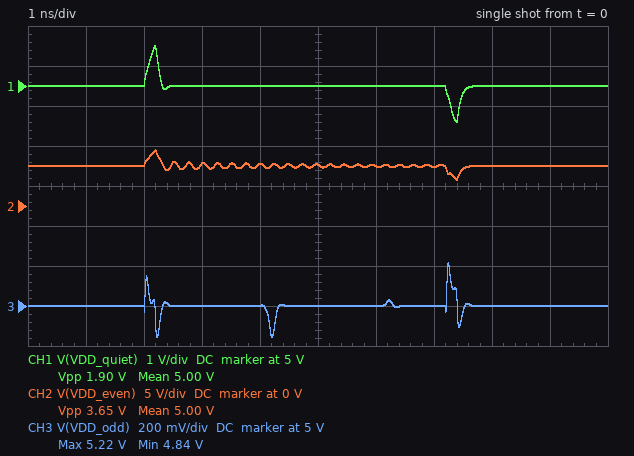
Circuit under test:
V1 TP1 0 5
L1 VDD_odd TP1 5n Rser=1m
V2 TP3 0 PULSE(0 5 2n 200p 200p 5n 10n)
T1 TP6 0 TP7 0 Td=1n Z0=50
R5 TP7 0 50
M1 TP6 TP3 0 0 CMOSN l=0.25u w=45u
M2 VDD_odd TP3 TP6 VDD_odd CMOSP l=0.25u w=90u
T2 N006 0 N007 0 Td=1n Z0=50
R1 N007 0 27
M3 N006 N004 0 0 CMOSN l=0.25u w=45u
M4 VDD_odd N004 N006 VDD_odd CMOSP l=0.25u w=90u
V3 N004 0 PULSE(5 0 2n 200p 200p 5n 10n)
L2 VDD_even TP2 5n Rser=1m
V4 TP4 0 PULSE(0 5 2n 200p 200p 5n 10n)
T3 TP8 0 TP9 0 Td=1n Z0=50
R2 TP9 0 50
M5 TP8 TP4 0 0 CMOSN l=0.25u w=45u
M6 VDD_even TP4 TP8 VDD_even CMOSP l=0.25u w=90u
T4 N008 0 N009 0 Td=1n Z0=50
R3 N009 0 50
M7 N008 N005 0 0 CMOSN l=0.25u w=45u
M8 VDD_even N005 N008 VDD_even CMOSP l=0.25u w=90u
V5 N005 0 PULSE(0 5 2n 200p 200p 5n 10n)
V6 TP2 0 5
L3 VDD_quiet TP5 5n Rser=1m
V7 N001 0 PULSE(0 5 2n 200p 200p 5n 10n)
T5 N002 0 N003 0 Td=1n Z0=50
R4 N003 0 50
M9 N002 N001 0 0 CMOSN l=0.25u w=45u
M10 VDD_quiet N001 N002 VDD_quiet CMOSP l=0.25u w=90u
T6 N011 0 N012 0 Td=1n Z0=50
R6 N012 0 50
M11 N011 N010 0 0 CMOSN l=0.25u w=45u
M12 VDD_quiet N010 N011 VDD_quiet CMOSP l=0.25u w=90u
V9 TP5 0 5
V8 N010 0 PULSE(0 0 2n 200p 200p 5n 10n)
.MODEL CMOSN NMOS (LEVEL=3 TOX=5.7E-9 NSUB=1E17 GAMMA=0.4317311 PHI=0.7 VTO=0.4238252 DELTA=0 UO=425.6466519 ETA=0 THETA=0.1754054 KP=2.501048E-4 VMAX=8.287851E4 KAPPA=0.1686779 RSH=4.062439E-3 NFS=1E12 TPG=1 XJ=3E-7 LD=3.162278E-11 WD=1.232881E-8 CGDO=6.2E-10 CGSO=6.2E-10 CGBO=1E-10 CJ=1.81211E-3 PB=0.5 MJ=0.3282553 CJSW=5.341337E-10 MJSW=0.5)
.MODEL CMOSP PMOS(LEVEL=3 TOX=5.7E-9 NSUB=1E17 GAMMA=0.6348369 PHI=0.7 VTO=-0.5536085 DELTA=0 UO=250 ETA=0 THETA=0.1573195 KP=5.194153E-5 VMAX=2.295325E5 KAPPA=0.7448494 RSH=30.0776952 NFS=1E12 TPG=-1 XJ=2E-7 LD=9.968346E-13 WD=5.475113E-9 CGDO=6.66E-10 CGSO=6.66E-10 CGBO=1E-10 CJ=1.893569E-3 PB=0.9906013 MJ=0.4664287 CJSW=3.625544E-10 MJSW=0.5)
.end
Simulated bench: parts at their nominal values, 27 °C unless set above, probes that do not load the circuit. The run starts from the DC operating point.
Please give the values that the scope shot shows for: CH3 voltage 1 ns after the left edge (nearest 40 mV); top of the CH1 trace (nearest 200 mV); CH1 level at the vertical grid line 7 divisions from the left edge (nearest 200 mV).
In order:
5.00 V
6.0 V
5.0 V
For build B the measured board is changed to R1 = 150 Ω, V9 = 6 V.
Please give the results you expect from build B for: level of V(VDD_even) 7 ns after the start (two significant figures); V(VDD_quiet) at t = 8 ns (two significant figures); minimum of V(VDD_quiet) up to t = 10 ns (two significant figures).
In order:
4.9 V
6.0 V
5.0 V
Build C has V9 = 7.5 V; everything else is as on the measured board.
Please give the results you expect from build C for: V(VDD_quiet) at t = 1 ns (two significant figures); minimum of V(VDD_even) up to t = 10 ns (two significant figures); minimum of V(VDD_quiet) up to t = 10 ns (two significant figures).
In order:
7.5 V
3.3 V
6.6 V
